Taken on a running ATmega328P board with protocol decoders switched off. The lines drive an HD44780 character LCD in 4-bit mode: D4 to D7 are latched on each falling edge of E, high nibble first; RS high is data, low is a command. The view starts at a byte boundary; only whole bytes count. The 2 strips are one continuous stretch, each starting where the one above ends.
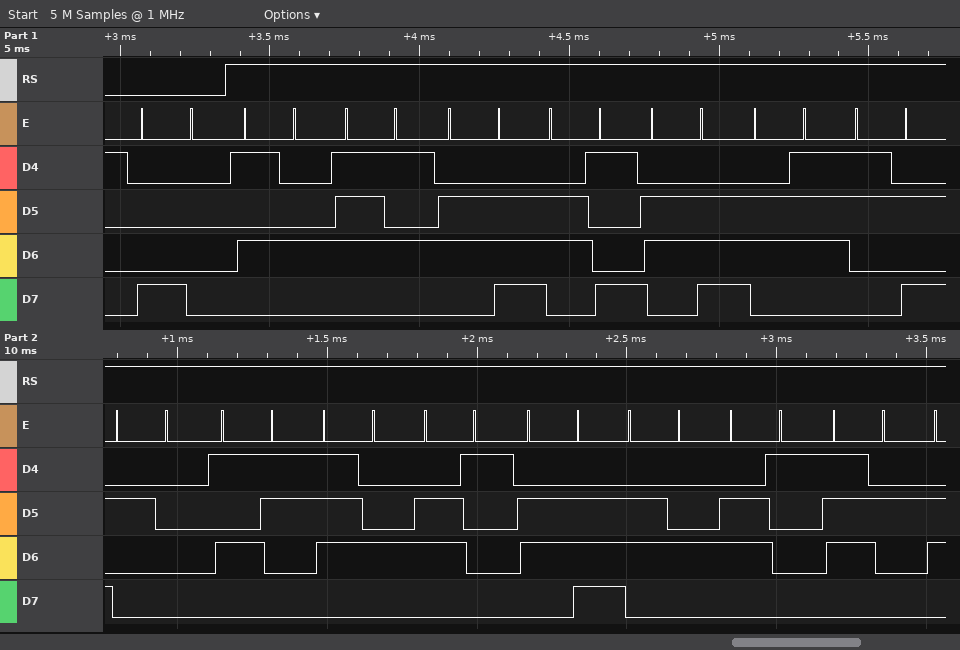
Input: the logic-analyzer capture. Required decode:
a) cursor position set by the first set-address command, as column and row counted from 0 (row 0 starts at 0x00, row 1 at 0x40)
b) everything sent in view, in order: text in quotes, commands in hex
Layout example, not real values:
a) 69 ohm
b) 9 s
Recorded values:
a) column 0, row 0
b) 0x80 "Tuning: Standar"
